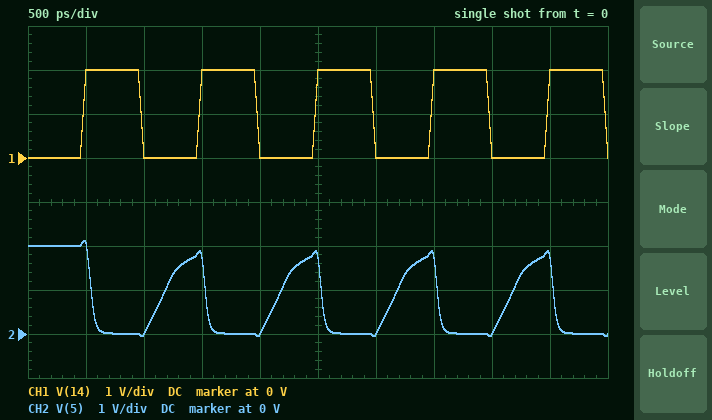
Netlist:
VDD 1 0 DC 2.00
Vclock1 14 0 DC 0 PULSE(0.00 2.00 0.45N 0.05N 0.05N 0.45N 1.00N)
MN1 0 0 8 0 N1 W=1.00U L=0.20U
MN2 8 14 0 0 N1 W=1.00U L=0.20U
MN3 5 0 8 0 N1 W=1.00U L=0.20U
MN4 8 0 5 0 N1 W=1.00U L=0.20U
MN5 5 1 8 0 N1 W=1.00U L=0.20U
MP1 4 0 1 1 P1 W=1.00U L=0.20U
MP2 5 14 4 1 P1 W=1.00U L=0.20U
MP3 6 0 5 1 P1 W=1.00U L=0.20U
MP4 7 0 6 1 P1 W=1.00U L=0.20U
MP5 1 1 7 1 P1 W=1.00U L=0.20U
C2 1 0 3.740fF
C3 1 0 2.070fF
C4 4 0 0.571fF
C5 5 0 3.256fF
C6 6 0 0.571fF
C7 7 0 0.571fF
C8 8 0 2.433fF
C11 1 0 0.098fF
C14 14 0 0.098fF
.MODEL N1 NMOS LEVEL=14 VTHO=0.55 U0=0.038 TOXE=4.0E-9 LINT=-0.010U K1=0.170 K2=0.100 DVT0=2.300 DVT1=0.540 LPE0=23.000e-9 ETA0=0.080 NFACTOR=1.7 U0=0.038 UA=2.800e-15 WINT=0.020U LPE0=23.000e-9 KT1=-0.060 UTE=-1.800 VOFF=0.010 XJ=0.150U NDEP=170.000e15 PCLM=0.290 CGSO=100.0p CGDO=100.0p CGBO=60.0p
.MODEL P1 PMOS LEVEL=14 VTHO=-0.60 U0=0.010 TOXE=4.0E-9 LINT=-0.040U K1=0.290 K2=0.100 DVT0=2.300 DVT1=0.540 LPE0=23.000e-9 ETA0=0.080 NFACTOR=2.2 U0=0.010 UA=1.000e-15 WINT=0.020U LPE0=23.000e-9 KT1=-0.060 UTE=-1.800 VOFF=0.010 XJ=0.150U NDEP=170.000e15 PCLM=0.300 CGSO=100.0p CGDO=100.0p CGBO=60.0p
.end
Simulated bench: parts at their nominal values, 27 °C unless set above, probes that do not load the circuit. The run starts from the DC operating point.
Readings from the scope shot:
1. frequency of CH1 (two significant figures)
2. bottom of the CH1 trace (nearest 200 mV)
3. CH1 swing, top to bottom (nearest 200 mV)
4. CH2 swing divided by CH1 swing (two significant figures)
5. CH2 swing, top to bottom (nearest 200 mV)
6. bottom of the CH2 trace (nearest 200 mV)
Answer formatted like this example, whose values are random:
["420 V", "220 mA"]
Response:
["1.0 GHz", "0 V", "2.0 V", "1.1", "2.2 V", "0 V"]
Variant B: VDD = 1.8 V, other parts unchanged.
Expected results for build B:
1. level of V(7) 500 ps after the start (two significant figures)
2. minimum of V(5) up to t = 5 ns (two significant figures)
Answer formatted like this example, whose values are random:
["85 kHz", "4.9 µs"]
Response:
["1.9 V", "-58 mV"]
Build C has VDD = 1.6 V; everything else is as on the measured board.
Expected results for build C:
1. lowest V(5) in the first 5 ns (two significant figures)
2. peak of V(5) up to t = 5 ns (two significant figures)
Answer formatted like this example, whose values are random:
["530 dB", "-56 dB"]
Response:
["-65 mV", "1.7 V"]
